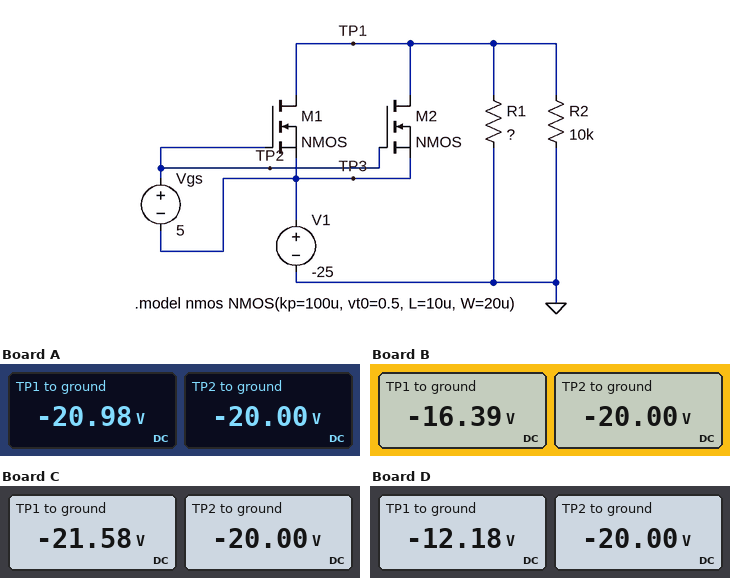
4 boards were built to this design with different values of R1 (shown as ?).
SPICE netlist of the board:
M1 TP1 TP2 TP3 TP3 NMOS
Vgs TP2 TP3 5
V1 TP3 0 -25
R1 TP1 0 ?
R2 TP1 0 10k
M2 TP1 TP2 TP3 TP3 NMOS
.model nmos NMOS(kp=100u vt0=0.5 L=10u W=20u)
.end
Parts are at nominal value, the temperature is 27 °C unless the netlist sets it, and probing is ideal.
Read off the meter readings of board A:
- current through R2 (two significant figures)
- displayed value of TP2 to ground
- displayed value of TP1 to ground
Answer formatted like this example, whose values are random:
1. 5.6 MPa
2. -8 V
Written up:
1. 2.1 mA
2. -20.00 V
3. -20.98 V
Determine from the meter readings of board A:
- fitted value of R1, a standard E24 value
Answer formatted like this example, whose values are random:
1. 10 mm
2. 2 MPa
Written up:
1. 11 kΩ
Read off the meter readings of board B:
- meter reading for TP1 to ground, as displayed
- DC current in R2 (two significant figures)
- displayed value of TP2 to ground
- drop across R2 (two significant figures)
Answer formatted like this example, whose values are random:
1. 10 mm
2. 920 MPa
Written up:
1. -16.39 V
2. 1.6 mA
3. -20.00 V
4. 16 V
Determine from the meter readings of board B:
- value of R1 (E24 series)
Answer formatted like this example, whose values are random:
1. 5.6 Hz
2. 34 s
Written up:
1. 6.8 kΩ
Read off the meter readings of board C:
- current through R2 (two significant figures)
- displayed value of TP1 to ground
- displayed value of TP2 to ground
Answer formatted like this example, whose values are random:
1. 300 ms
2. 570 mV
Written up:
1. 2.2 mA
2. -21.58 V
3. -20.00 V
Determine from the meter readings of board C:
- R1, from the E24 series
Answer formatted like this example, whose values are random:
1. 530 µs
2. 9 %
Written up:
1. 13 kΩ
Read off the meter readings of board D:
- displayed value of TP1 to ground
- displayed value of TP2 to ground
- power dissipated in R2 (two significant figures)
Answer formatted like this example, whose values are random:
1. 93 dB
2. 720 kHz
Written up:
1. -12.18 V
2. -20.00 V
3. 15 mW
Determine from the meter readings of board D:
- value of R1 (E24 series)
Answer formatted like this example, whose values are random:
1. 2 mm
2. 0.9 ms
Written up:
1. 4.3 kΩ
